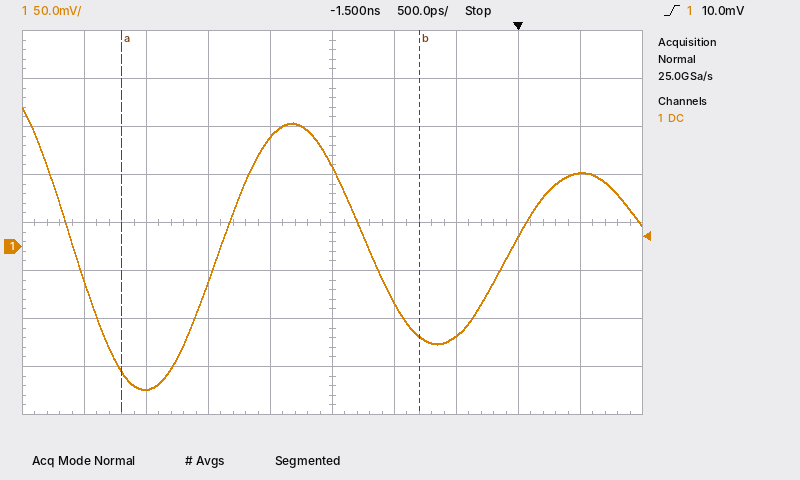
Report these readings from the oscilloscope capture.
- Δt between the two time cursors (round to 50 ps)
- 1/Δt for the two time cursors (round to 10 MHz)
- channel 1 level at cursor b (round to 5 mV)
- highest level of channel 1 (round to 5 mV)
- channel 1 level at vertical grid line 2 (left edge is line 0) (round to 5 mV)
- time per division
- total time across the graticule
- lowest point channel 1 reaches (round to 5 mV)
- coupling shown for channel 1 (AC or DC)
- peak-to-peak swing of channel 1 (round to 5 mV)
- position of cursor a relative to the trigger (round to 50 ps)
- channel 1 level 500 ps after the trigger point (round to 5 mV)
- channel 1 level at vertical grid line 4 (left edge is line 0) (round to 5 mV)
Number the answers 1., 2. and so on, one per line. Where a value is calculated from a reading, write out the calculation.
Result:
1. 2.40 ns
2. 1 / 2.40 ns ≈ 420 MHz
3. -95 mV
4. 145 mV
5. -150 mV
6. 500 ps
7. 5 ns
8. -150 mV
9. DC
10. 145 mV − (-150 mV) = 295 mV
11. -3.20 ns
12. 75 mV
13. 115 mV
